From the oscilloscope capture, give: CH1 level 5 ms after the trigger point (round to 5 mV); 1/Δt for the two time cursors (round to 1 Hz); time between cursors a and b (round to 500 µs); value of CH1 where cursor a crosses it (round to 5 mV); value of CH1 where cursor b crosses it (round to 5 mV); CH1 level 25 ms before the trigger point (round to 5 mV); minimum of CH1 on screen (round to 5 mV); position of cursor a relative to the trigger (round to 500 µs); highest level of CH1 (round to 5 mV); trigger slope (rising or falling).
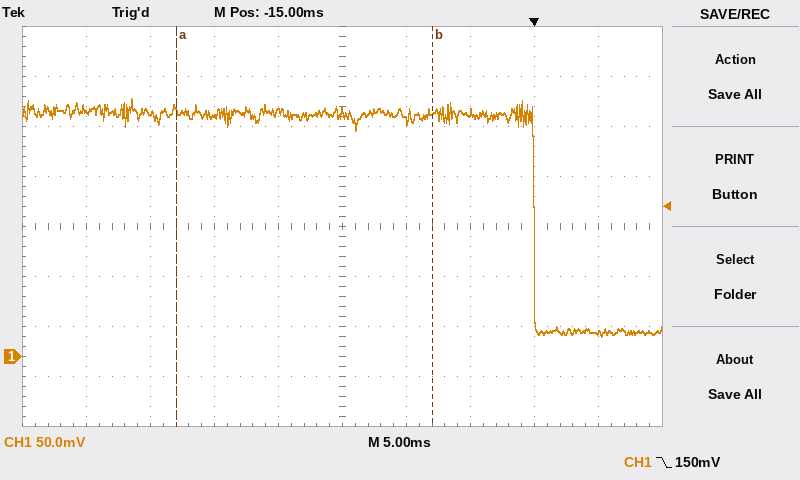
25 mV
50 Hz
20.0 ms
245 mV
245 mV
240 mV
20 mV
-28.0 ms
260 mV
falling
